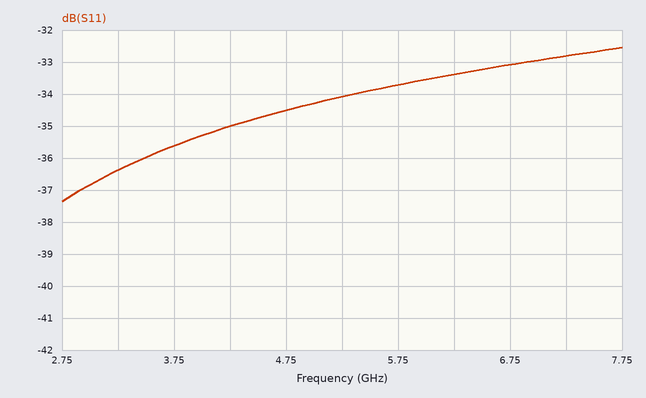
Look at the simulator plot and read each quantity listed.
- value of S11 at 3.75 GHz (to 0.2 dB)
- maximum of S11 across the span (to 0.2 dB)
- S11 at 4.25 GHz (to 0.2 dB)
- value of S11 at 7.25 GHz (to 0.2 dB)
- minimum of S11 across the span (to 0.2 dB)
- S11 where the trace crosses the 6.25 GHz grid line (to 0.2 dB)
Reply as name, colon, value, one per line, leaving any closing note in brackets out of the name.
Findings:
value of S11 at 3.75 GHz: -35.6 dB
maximum of S11 across the span: -32.6 dB
S11 at 4.25 GHz: -35.0 dB
value of S11 at 7.25 GHz: -32.8 dB
minimum of S11 across the span: -37.4 dB
S11 where the trace crosses the 6.25 GHz grid line: -33.4 dB
